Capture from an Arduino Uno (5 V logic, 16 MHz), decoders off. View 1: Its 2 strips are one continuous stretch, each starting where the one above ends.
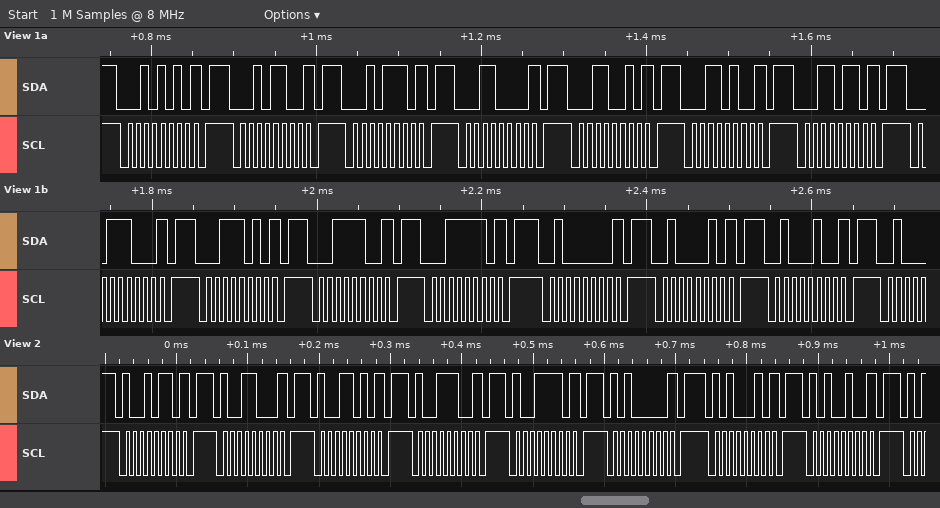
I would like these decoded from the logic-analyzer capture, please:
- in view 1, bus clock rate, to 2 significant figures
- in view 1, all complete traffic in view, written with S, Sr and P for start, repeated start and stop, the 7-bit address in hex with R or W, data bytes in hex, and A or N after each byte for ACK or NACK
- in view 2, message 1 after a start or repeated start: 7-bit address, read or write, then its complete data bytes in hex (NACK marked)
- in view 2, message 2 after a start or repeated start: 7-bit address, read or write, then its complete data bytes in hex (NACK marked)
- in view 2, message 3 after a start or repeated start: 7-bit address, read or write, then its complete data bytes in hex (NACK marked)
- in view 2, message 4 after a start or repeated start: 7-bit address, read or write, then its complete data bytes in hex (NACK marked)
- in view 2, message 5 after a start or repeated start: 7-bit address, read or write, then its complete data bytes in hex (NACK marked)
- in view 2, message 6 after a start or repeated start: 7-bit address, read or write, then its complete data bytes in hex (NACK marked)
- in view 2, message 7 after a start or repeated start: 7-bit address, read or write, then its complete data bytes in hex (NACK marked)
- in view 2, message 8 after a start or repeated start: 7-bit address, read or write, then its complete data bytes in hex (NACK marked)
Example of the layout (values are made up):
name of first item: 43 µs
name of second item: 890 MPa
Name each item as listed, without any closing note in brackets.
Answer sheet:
in view 1, bus clock rate, to 2 significant figures: 100 kHz
in view 1, all complete traffic in view, written with S, Sr and P for start, repeated start and stop, the 7-bit address in hex with R or W, data bytes in hex, and A or N after each byte for ACK or NACK: S 15W N P S 16W N P S 17W N P S 18W N P S 19W N P S 1AW N P S 1BW N P S 1CW N P S 1DW N P S 1EW N P S 1FW N P S 20W N P S 21W N P S 22W N P
in view 2, message 1 after a start or repeated start: 7-bit address, read or write, then its complete data bytes in hex: 0x4B write NACK
in view 2, message 2 after a start or repeated start: 7-bit address, read or write, then its complete data bytes in hex: 0x4C write NACK
in view 2, message 3 after a start or repeated start: 7-bit address, read or write, then its complete data bytes in hex: 0x4D write NACK
in view 2, message 4 after a start or repeated start: 7-bit address, read or write, then its complete data bytes in hex: 0x4E write NACK
in view 2, message 5 after a start or repeated start: 7-bit address, read or write, then its complete data bytes in hex: 0x4F write NACK
in view 2, message 6 after a start or repeated start: 7-bit address, read or write, then its complete data bytes in hex: 0x50 write NACK
in view 2, message 7 after a start or repeated start: 7-bit address, read or write, then its complete data bytes in hex: 0x51 write NACK
in view 2, message 8 after a start or repeated start: 7-bit address, read or write, then its complete data bytes in hex: 0x52 write NACK
